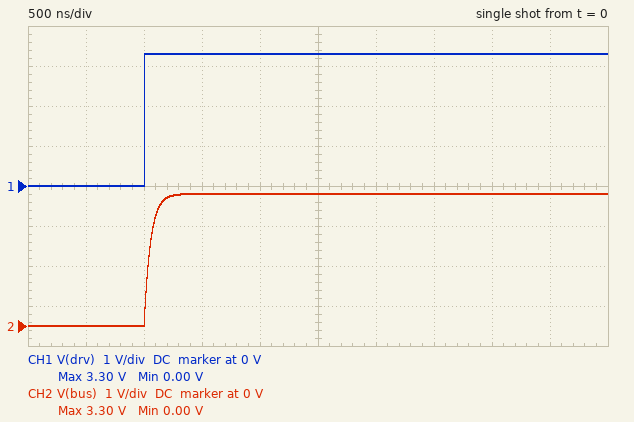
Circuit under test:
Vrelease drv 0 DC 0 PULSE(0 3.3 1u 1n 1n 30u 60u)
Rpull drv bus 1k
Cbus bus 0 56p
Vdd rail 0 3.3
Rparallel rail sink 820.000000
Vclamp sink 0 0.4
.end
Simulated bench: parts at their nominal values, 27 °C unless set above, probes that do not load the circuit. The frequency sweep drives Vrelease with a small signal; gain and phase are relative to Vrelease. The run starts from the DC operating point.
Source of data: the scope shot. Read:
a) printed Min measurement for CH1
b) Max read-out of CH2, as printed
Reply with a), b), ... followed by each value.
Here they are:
a) 0.00 V
b) 3.30 V
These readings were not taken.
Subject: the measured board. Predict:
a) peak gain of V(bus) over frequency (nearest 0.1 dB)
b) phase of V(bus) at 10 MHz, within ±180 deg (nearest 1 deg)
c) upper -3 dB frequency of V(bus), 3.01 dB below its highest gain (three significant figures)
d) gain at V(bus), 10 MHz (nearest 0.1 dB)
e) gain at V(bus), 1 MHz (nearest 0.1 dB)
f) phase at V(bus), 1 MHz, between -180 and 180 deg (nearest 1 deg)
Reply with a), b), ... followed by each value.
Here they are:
a) 0 dB
b) -74 deg
c) 2.84 MHz
d) -11.3 dB
e) -0.5 dB
f) -19 deg
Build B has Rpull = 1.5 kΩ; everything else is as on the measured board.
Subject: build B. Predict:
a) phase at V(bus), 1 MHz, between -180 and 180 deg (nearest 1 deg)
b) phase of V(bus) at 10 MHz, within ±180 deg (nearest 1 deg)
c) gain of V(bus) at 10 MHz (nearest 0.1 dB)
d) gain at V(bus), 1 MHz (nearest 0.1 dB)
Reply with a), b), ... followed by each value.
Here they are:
a) -28 deg
b) -79 deg
c) -14.6 dB
d) -1.1 dB
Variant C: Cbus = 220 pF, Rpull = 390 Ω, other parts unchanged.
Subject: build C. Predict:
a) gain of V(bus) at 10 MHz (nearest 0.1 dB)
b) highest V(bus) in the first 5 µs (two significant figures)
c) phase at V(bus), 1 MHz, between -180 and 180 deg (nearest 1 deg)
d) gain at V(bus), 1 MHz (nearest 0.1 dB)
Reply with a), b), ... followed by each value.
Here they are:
a) -14.8 dB
b) 3.3 V
c) -28 deg
d) -1.1 dB
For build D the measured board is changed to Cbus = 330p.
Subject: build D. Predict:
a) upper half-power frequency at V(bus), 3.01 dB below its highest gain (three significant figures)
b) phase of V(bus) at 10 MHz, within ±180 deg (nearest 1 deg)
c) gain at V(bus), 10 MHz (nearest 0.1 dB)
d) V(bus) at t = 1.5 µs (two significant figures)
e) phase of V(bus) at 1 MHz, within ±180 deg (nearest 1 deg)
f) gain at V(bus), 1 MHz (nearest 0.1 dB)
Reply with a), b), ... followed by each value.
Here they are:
a) 482 kHz
b) -87 deg
c) -26.3 dB
d) 2.6 V
e) -64 deg
f) -7.2 dB
